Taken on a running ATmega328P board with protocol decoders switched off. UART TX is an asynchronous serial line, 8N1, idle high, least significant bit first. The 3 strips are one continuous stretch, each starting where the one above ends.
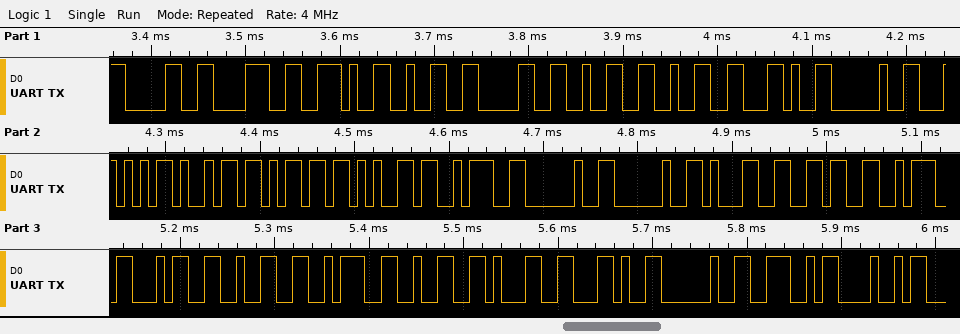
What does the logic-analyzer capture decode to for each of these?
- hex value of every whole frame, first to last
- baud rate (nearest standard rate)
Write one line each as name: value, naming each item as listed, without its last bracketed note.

hex value of every whole frame, first to last: 30 38 2E 32 30 32 32 2C 20 54 69 6D 65 3A 20 20 31 36 3A 34 32 3A 32 31 2C 20 4E 48
baud rate: 115200 baud
